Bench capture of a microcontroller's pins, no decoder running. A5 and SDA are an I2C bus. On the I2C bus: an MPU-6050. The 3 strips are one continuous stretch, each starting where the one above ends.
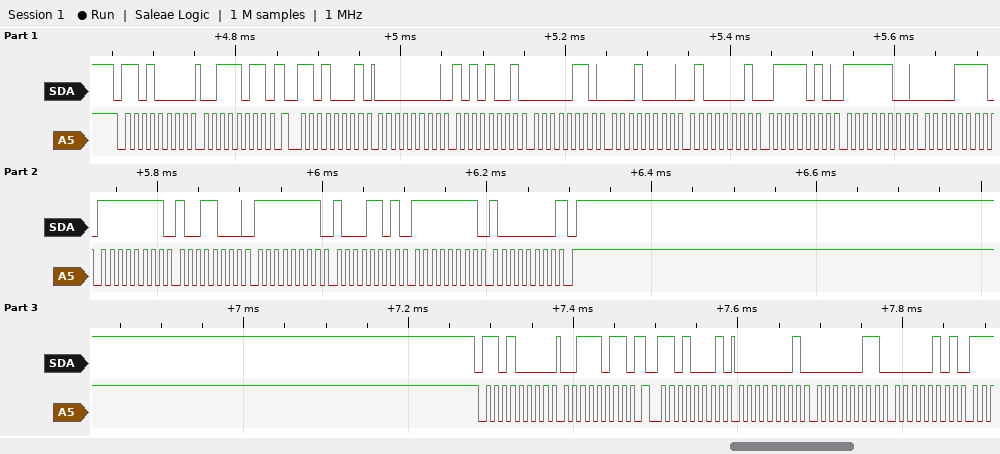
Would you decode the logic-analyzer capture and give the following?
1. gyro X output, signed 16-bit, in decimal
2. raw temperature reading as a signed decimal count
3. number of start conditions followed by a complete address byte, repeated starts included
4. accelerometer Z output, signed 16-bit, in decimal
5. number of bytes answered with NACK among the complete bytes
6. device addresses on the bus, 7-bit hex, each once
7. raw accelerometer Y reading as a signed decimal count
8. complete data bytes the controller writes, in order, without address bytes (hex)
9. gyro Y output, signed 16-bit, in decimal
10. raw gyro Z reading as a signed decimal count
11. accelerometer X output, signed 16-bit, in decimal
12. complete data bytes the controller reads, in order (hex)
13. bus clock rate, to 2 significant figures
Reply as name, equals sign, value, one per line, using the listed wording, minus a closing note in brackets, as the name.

gyro X output, signed 16-bit, in decimal = -104
raw temperature reading as a signed decimal count = -1009
number of start conditions followed by a complete address byte, repeated starts included = 4
accelerometer Z output, signed 16-bit, in decimal = 16762
number of bytes answered with NACK among the complete bytes = 1
device addresses on the bus, 7-bit hex, each once = 0x68
raw accelerometer Y reading as a signed decimal count = 1552
complete data bytes the controller writes, in order, without address bytes = 3B 3B
gyro Y output, signed 16-bit, in decimal = -115
raw gyro Z reading as a signed decimal count = -128
accelerometer X output, signed 16-bit, in decimal = 169
complete data bytes the controller reads, in order = 00 A9 06 10 41 7A FC 0F FF 98 FF 8D FF 80 01 03 05
bus clock rate, to 2 significant figures = 100 kHz
